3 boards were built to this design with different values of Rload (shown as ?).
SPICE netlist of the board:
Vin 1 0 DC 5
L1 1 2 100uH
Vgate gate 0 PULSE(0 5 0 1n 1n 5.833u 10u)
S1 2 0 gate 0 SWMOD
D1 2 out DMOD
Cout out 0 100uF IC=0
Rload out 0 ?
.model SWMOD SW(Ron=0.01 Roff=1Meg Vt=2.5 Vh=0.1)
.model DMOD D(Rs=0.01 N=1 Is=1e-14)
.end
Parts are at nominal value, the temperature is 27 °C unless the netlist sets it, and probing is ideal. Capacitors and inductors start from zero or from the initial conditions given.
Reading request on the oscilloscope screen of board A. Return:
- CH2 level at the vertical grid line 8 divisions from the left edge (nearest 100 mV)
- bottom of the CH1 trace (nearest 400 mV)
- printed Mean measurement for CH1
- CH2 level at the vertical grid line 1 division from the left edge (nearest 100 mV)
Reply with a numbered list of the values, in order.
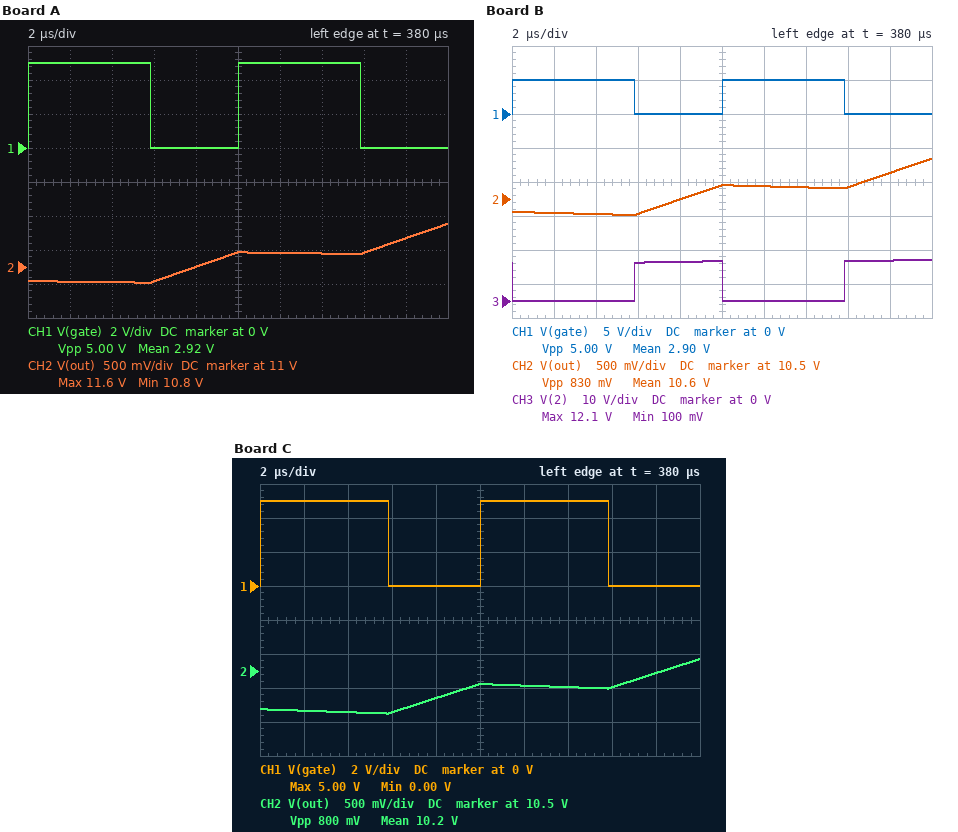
1. 11.2 V
2. 0 V
3. 2.92 V
4. 10.8 V
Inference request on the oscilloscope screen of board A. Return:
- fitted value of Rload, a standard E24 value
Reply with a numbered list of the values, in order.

1. 27 Ω
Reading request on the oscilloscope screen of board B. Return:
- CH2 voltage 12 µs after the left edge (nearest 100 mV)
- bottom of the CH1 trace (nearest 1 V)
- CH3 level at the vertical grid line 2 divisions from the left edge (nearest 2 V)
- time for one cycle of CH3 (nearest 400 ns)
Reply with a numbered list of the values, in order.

1. 10.7 V
2. 0 V
3. 0 V
4. 10.0 µs
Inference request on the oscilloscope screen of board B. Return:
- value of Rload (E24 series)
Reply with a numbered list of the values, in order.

1. 13 Ω
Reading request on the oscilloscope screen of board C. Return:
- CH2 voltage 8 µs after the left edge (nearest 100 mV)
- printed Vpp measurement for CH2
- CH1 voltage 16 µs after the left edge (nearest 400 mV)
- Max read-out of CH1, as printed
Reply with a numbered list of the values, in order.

1. 10.1 V
2. 800 mV
3. 0 V
4. 5.00 V
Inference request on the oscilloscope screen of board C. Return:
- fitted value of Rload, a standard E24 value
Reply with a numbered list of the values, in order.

1. 9.1 Ω
